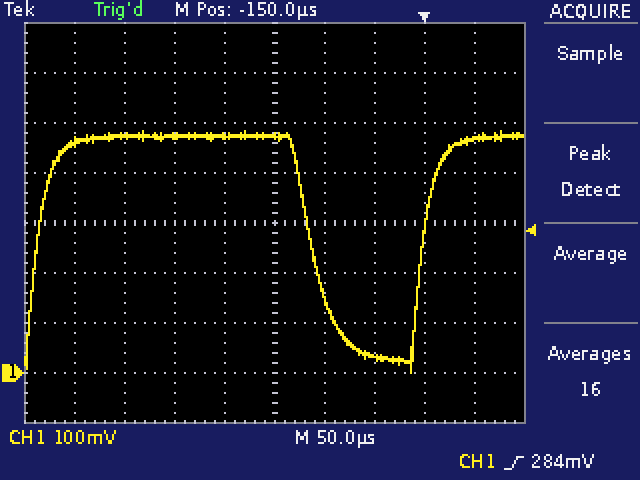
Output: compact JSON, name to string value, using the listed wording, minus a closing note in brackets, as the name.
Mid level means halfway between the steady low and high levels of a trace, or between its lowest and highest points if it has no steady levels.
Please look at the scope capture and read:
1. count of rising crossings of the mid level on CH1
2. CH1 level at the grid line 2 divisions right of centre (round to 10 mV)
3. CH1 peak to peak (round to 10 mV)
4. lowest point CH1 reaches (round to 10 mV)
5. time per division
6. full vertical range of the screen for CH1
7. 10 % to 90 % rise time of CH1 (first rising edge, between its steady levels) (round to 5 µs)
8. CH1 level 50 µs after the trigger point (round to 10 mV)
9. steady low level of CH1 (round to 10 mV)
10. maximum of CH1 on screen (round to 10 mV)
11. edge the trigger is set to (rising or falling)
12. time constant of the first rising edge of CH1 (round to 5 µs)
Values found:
{"count of rising crossings of the mid level on CH1": "2", "CH1 level at the grid line 2 divisions right of centre": "30 mV", "CH1 peak to peak": "480 mV", "lowest point CH1 reaches": "0 mV", "time per division": "50 µs", "full vertical range of the screen for CH1": "800 mV", "10 % to 90 % rise time of CH1 (first rising edge, between its steady levels)": "30 µs", "CH1 level 50 µs after the trigger point": "470 mV", "steady low level of CH1": "30 mV", "maximum of CH1 on screen": "480 mV", "edge the trigger is set to": "rising", "time constant of the first rising edge of CH1": "15 µs"}
